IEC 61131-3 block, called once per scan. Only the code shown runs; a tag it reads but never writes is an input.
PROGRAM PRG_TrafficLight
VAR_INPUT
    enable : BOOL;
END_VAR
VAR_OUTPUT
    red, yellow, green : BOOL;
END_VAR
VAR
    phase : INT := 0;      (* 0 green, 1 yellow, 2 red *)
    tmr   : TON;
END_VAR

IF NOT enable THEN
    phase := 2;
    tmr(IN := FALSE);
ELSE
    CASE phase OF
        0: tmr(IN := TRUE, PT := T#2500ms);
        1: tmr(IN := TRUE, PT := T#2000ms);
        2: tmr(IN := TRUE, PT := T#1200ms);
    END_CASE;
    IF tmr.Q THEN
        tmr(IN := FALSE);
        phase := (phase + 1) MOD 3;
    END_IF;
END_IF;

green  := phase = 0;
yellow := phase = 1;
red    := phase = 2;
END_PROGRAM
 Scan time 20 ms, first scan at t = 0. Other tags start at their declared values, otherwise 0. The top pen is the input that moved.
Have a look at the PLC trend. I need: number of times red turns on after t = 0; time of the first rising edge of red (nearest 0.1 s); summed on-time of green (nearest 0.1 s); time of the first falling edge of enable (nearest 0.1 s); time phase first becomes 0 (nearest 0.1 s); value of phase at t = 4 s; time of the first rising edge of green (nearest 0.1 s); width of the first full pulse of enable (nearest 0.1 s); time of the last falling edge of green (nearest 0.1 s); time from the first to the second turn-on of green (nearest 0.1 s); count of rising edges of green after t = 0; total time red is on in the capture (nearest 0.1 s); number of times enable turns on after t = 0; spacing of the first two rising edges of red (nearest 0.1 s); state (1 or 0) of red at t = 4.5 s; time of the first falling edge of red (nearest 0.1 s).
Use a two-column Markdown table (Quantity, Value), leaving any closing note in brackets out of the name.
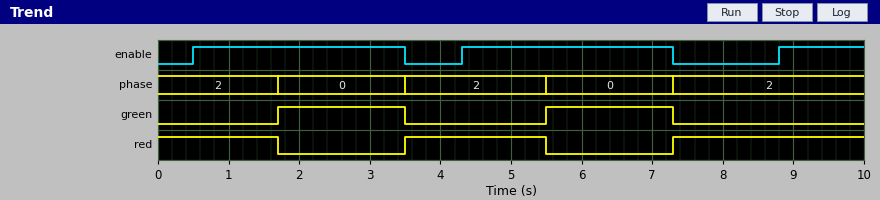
| Quantity | Value |
|---|---|
| number of times red turns on after t = 0 | 2 |
| time of the first rising edge of red | 3.5 s |
| summed on-time of green | 3.6 s |
| time of the first falling edge of enable | 3.5 s |
| time phase first becomes 0 | 1.7 s |
| value of phase at t = 4 s | 2 |
| time of the first rising edge of green | 1.7 s |
| width of the first full pulse of enable | 3.0 s |
| time of the last falling edge of green | 7.3 s |
| time from the first to the second turn-on of green | 3.8 s |
| count of rising edges of green after t = 0 | 2 |
| total time red is on in the capture | 6.4 s |
| number of times enable turns on after t = 0 | 3 |
| spacing of the first two rising edges of red | 3.8 s |
| state (1 or 0) of red at t = 4.5 s | 1 |
| time of the first falling edge of red | 1.7 s |
